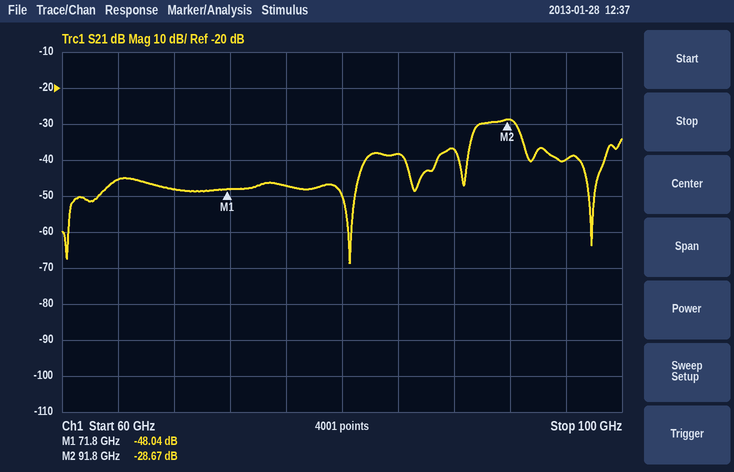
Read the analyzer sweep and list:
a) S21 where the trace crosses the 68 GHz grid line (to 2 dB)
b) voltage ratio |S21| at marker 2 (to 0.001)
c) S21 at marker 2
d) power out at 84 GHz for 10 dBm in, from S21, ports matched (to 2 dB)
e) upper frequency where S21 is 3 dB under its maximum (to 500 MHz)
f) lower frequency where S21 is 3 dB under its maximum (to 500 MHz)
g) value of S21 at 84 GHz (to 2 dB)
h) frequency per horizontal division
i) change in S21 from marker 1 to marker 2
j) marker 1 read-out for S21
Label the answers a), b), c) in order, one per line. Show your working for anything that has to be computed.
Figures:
a) -48 dB
b) 10^(-28.67/20) ≈ 0.037
c) -28.67 dB
d) 10 dBm + (-38 dB) = -28 dBm
e) 92.5 GHz
f) 89.5 GHz
g) -38 dB
h) 4 GHz
i) -28.67 − (-48.04) = 19.37 dB
j) -48.04 dB
